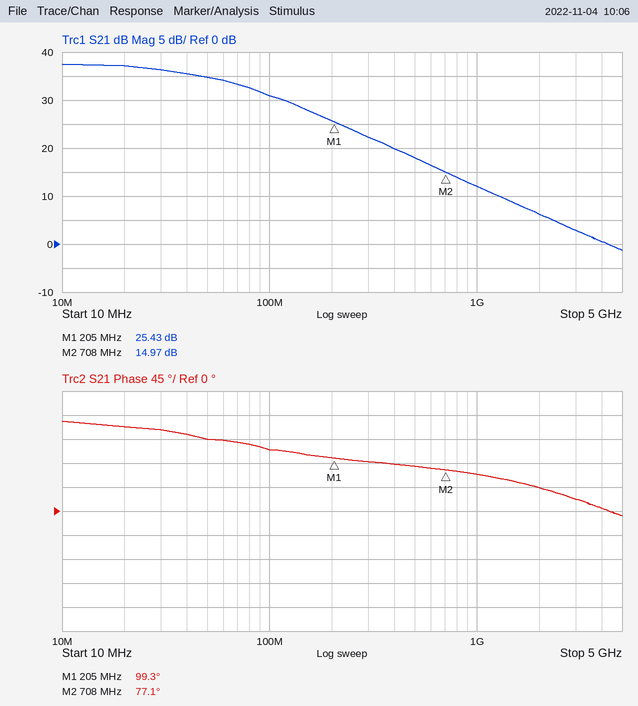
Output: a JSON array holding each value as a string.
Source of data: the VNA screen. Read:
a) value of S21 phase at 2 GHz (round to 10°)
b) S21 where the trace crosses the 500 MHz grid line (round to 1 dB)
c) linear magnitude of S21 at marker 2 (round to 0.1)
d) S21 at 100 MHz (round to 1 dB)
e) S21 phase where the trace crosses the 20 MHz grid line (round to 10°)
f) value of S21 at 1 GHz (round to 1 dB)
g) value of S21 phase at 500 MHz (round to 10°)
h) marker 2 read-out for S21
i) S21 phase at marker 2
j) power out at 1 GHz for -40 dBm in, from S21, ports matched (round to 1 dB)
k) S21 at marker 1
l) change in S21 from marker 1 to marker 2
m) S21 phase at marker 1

["40°", "18 dB", "5.6", "31 dB", "160°", "12 dB", "80°", "14.97 dB", "77.1°", "-28 dBm", "25.43 dB", "-10.46 dB", "99.3°"]
